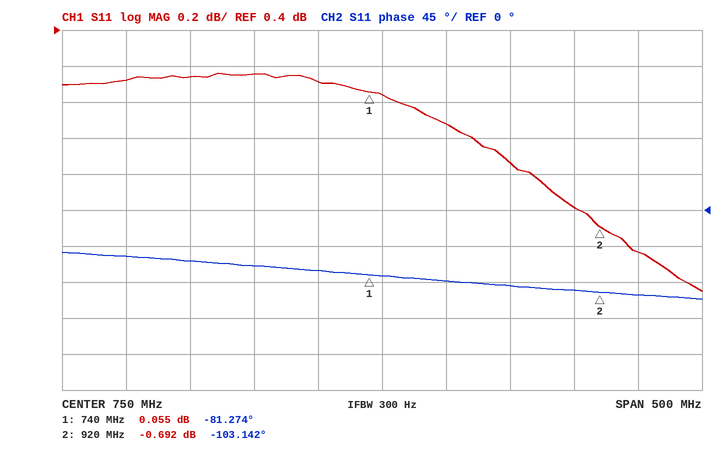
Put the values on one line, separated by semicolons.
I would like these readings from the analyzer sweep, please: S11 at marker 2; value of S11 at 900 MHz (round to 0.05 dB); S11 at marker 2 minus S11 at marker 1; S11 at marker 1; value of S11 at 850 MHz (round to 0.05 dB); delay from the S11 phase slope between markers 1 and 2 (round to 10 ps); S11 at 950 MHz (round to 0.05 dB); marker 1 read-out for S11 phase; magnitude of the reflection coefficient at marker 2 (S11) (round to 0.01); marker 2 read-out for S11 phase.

-0.692 dB; -0.60 dB; -0.747 dB; 0.055 dB; -0.35 dB; 340 ps; -0.85 dB; -81.274°; 0.92; -103.142°
